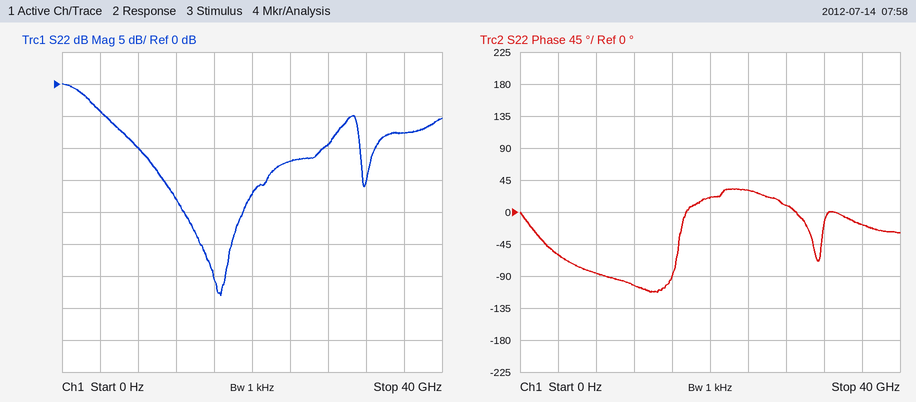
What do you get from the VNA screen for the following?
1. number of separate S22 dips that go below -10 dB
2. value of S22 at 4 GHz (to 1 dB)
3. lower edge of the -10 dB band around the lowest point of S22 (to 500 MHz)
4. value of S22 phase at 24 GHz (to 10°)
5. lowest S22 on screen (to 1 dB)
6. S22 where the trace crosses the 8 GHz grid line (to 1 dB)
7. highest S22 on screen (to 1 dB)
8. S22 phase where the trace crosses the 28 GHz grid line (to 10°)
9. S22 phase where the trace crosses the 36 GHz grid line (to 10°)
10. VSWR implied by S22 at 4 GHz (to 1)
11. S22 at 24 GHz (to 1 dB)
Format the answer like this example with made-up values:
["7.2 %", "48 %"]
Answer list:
["2", "-4 dB", "8.0 GHz", "30°", "-33 dB", "-10 dB", "0 dB", "10°", "-20°", "4", "-12 dB"]
